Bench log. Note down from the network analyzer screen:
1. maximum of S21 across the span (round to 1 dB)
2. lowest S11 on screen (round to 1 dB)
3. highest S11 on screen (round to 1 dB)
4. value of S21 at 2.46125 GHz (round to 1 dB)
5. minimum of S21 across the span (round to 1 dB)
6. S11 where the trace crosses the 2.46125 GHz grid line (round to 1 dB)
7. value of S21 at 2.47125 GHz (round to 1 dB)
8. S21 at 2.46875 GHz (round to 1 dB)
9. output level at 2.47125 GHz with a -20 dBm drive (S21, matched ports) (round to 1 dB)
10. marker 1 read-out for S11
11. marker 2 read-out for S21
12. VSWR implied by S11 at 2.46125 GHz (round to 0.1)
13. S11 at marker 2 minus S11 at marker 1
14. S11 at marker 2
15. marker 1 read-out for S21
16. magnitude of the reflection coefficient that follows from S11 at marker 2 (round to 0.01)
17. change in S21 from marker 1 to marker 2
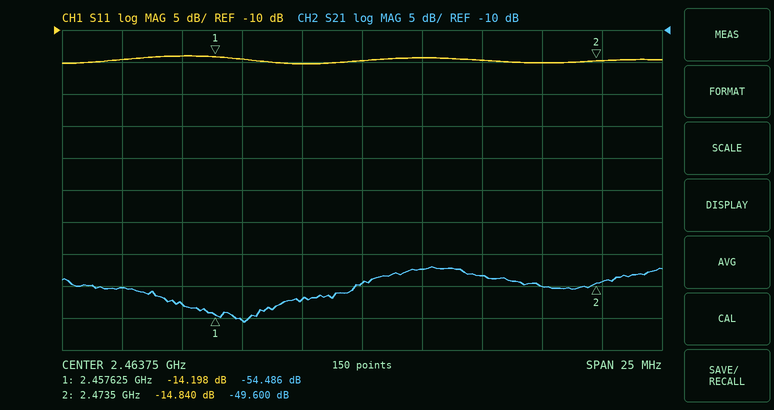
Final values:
-47 dB
-15 dB
-14 dB
-52 dB
-56 dB
-15 dB
-50 dB
-48 dB
-70 dBm
-14.198 dB
-49.600 dB
1.4
-0.642 dB
-14.840 dB
-54.486 dB
0.18
4.886 dB
